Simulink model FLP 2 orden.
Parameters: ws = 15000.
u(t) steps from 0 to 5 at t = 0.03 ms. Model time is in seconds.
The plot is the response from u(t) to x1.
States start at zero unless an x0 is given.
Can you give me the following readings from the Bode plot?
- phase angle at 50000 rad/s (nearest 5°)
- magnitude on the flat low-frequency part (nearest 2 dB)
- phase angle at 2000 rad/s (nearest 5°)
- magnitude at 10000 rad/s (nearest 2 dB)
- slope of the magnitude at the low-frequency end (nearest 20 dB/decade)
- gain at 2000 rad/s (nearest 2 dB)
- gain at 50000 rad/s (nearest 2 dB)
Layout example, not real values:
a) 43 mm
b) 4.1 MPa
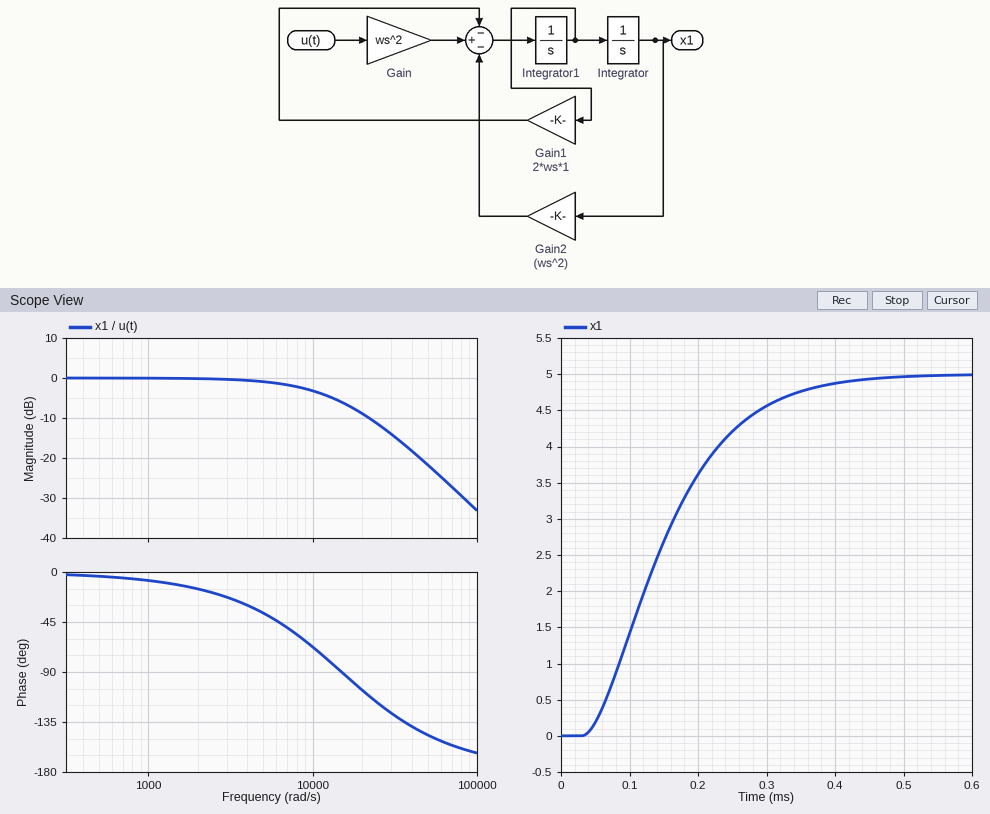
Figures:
a) -145°
b) 0 dB
c) -15°
d) -4 dB
e) 0 dB/decade
f) 0 dB
g) -22 dB
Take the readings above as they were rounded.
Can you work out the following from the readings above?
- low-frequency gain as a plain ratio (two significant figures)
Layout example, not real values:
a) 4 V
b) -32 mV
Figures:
a) 1.0
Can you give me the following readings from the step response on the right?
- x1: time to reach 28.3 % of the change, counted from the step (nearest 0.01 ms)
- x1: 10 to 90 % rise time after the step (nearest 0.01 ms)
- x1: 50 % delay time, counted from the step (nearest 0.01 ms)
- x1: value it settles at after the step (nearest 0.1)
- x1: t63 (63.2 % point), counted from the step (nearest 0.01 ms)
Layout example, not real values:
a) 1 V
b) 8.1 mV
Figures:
a) 0.07 ms
b) 0.22 ms
c) 0.11 ms
d) 5.0
e) 0.14 ms
